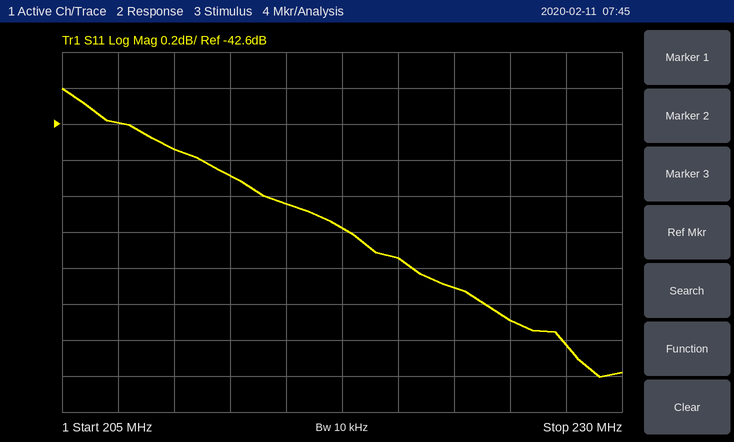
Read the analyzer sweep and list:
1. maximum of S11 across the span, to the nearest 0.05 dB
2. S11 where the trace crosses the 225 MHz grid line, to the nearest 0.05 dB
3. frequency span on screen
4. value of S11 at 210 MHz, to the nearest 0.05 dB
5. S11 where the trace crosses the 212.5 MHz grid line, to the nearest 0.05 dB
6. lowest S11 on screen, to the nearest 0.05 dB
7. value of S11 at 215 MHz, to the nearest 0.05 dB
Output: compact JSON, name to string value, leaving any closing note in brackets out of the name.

{"maximum of S11 across the span, to the nearest 0.05 dB": "-42.40 dB", "S11 where the trace crosses the 225 MHz grid line, to the nearest 0.05 dB": "-43.70 dB", "frequency span on screen": "25 MHz", "value of S11 at 210 MHz, to the nearest 0.05 dB": "-42.75 dB", "S11 where the trace crosses the 212.5 MHz grid line, to the nearest 0.05 dB": "-42.90 dB", "lowest S11 on screen, to the nearest 0.05 dB": "-44.00 dB", "value of S11 at 215 MHz, to the nearest 0.05 dB": "-43.05 dB"}
